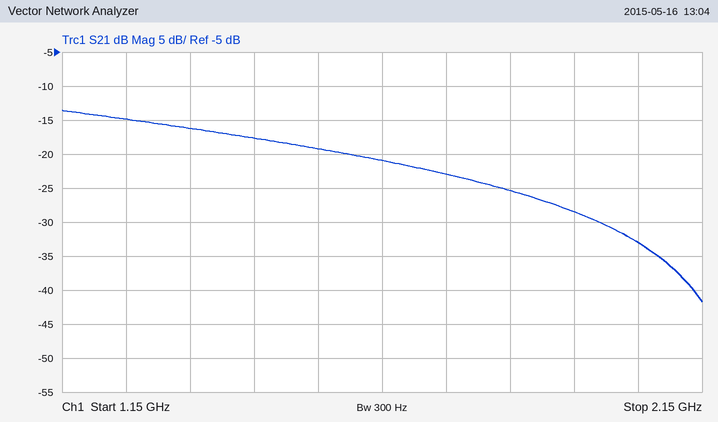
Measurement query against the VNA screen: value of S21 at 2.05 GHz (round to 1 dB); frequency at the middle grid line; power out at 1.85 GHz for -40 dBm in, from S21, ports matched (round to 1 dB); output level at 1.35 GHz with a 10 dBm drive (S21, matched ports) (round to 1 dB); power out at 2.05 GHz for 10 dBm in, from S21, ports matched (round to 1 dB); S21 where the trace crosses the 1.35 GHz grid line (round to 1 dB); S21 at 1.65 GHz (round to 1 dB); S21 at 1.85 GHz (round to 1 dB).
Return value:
-33 dB
1.65 GHz
-65 dBm
-6 dBm
-23 dBm
-16 dB
-21 dB
-25 dB
